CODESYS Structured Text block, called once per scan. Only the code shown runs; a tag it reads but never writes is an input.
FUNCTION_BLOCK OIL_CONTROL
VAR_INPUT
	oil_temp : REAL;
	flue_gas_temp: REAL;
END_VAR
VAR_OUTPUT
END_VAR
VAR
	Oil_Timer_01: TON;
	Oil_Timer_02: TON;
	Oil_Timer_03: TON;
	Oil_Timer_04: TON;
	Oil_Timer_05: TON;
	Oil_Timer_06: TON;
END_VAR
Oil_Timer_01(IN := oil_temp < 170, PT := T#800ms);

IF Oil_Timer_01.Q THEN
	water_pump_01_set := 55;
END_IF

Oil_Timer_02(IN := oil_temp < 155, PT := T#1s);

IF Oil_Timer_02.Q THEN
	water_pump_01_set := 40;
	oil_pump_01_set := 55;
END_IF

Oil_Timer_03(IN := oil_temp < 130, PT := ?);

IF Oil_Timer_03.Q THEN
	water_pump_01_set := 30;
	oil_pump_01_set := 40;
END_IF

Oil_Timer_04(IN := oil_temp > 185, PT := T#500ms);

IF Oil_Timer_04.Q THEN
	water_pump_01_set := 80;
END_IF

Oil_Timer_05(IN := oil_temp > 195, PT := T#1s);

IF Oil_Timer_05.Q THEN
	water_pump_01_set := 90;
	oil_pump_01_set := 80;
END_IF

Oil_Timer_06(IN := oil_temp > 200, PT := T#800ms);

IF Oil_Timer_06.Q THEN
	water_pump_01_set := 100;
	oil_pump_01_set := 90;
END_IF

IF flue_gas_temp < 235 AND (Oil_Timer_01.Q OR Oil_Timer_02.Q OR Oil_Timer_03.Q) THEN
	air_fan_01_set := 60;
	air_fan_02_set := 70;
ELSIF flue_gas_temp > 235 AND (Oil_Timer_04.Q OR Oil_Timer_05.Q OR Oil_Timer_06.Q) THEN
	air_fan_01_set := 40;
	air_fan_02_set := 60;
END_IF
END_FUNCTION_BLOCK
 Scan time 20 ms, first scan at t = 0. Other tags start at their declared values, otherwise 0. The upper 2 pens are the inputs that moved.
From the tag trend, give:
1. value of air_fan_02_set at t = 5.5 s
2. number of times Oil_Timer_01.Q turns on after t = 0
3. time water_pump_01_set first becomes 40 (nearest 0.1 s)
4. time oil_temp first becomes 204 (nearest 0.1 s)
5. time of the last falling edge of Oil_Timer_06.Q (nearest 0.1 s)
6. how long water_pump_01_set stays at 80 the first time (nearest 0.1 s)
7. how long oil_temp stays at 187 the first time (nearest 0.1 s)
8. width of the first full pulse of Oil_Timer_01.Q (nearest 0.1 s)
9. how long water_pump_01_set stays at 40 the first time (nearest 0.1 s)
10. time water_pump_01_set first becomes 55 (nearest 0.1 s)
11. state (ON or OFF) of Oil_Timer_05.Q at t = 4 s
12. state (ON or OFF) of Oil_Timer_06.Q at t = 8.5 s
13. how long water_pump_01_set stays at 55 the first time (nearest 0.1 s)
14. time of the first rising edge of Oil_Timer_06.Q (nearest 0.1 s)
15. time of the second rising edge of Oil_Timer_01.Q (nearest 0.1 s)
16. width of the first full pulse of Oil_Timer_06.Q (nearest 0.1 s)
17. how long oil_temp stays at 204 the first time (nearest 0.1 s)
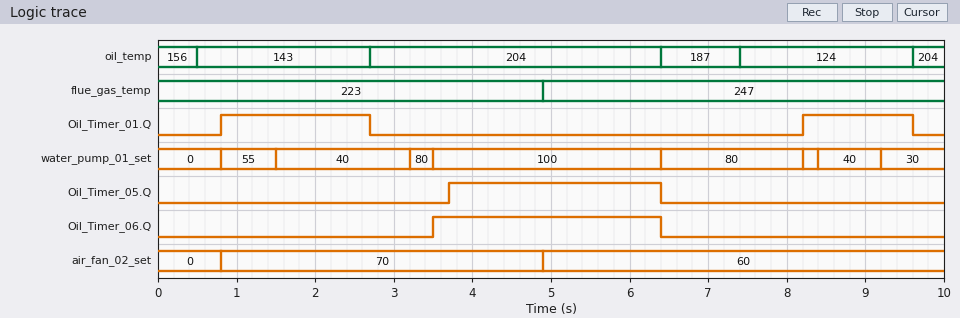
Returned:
60
2
1.5 s
2.7 s
6.4 s
0.3 s
1.0 s
1.9 s
1.7 s
0.8 s
ON
OFF
0.7 s
3.5 s
8.2 s
2.9 s
3.7 s
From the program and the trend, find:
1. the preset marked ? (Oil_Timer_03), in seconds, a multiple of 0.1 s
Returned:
1.8 s
